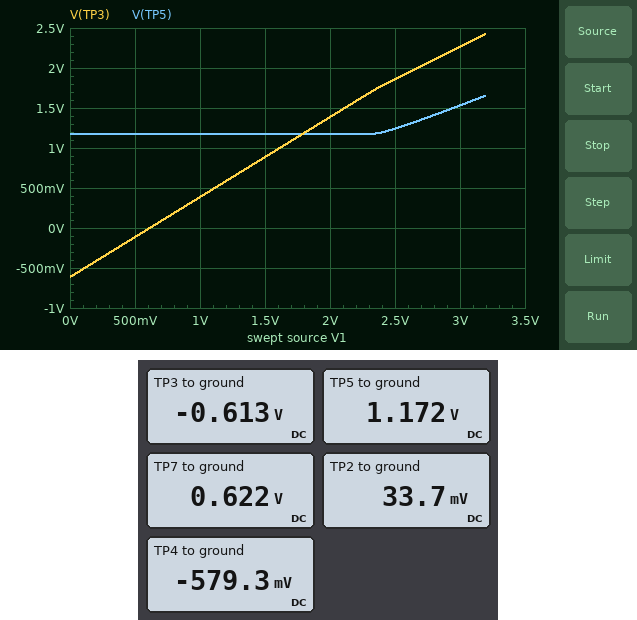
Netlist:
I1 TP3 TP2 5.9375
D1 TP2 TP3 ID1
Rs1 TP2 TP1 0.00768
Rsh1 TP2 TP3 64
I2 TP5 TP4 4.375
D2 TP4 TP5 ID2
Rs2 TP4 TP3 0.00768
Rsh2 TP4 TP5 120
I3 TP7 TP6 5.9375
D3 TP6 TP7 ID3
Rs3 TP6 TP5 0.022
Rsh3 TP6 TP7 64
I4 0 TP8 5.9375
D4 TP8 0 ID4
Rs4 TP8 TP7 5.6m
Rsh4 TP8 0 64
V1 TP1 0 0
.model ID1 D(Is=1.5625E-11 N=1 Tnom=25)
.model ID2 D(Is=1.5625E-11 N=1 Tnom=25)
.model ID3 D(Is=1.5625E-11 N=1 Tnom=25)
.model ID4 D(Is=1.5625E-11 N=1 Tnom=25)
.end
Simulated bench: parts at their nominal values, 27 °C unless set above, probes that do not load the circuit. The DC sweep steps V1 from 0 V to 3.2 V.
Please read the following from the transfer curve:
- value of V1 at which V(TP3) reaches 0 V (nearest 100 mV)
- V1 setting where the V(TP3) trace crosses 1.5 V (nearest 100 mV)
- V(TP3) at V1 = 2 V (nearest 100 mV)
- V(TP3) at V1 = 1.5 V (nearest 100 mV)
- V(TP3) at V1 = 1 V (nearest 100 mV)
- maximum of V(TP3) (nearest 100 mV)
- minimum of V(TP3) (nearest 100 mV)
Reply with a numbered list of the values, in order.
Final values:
1. 600 mV
2. 2.1 V
3. 1.4 V
4. 900 mV
5. 400 mV
6. 2.4 V
7. -600 mV
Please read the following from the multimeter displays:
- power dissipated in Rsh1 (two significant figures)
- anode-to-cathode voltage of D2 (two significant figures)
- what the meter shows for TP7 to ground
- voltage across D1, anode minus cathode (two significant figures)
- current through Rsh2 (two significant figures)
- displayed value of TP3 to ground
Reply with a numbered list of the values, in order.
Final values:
1. 6.5 mW
2. -1.8 V
3. 0.622 V
4. 650 mV
5. 15 mA
6. -0.613 V
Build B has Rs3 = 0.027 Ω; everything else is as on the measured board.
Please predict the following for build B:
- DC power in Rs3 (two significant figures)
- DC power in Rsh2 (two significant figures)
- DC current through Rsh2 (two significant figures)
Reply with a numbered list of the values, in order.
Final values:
1. 520 mW
2. 25 mW
3. 14 mA
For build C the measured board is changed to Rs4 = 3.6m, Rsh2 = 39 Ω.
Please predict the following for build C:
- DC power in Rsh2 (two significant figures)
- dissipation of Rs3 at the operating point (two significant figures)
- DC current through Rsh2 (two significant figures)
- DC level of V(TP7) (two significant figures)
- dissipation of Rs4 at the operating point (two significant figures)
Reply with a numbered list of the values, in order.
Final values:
1. 79 mW
2. 430 mW
3. 45 mA
4. 630 mV
5. 70 mW
